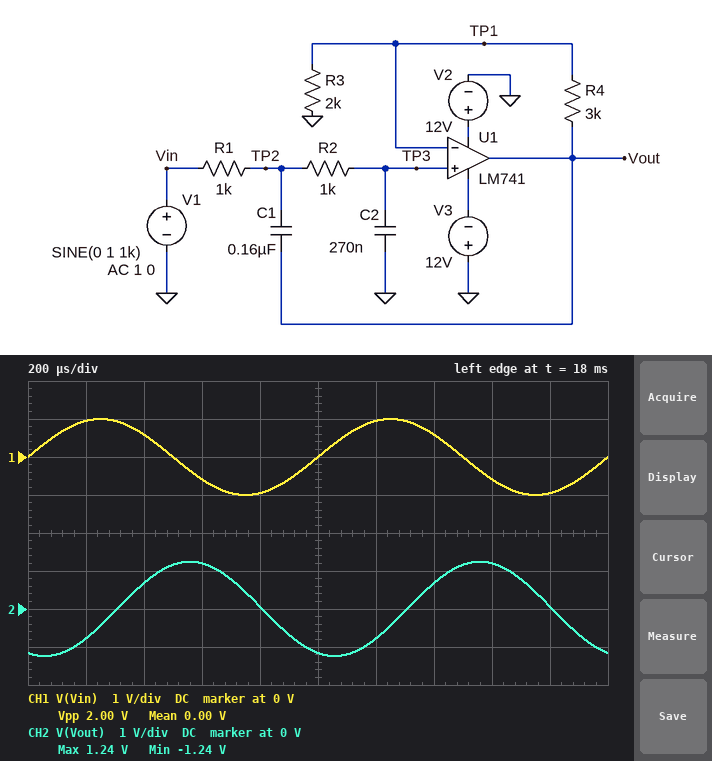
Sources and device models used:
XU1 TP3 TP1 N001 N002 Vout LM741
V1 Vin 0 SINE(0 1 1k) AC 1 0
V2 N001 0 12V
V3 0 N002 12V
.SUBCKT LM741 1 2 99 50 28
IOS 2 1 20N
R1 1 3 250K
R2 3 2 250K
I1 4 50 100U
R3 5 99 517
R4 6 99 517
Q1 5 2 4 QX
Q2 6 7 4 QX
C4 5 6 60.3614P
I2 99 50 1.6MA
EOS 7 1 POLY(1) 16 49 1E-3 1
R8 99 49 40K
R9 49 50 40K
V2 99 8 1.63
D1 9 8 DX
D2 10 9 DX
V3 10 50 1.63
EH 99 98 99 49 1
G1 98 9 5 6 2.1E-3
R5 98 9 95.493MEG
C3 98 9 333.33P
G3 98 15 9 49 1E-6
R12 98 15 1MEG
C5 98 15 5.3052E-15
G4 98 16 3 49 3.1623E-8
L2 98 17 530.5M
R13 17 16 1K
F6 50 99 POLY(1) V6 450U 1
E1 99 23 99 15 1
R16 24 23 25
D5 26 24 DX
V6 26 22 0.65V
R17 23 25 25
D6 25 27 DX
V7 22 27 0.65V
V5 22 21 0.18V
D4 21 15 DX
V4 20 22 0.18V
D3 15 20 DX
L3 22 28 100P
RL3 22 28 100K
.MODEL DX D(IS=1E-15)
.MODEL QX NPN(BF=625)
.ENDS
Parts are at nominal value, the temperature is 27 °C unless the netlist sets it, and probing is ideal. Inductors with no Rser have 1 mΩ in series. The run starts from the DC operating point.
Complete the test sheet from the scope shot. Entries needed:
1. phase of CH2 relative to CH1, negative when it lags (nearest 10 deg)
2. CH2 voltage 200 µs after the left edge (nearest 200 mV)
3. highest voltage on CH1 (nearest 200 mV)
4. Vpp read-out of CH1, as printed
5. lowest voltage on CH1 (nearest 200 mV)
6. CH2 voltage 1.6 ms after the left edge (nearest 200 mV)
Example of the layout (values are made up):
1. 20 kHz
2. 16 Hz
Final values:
1. -110 deg
2. -800 mV
3. 1.0 V
4. 2.00 V
5. -1.0 V
6. 1.2 V
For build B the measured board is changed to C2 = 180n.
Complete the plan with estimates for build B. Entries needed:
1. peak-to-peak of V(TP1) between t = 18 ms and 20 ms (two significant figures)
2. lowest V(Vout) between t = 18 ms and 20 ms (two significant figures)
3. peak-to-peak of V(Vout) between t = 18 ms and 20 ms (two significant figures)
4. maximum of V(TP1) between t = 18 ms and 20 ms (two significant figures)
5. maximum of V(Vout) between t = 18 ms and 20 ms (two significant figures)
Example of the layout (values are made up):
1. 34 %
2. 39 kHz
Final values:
1. 2.6 V
2. -3.3 V
3. 6.5 V
4. 1.3 V
5. 3.3 V
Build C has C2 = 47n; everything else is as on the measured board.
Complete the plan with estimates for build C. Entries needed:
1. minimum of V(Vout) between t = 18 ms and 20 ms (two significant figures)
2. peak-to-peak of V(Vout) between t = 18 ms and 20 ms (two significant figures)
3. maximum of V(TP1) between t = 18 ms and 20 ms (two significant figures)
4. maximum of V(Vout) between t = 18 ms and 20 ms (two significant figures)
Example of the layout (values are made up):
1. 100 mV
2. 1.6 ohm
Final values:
1. -11 V
2. 22 V
3. 4.3 V
4. 11 V
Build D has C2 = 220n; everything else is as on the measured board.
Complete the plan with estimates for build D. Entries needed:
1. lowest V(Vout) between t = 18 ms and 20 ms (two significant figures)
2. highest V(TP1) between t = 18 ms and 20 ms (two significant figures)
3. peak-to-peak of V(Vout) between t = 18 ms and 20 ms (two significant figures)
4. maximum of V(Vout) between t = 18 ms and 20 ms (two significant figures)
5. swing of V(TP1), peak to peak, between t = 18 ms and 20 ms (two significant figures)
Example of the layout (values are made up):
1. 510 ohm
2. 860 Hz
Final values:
1. -1.9 V
2. 760 mV
3. 3.8 V
4. 1.9 V
5. 1.5 V
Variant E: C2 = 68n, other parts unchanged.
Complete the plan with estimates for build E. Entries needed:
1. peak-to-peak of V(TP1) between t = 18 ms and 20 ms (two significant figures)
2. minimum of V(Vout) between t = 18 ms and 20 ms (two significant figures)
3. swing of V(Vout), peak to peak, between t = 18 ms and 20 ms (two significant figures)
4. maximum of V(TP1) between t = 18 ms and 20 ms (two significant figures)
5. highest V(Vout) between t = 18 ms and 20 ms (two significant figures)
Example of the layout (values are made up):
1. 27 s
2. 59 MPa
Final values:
1. 8.7 V
2. -11 V
3. 22 V
4. 4.3 V
5. 11 V
